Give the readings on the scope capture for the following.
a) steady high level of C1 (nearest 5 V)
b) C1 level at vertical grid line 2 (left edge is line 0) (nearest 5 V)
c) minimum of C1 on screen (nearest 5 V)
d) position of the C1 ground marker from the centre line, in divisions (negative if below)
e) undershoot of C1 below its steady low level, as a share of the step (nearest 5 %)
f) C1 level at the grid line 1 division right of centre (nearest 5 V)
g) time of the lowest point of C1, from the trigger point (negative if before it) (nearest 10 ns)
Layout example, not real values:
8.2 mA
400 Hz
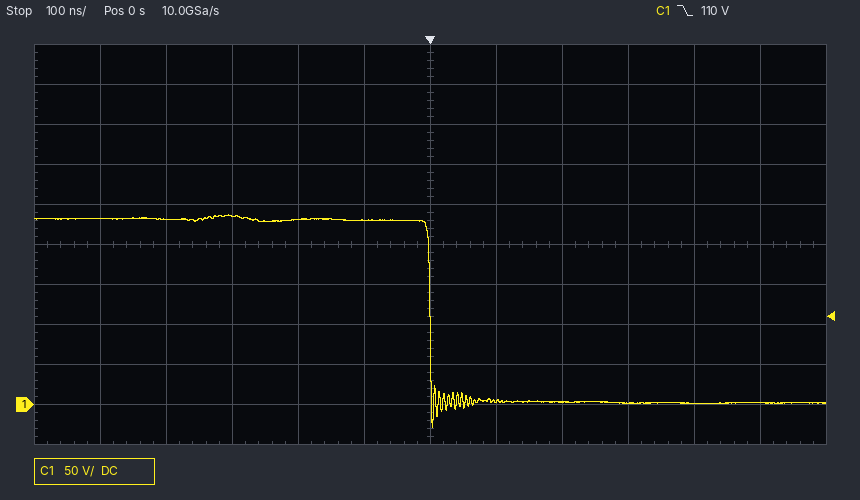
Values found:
230 V
230 V
-30 V
-4.0 div
15 %
5 V
0 ns
